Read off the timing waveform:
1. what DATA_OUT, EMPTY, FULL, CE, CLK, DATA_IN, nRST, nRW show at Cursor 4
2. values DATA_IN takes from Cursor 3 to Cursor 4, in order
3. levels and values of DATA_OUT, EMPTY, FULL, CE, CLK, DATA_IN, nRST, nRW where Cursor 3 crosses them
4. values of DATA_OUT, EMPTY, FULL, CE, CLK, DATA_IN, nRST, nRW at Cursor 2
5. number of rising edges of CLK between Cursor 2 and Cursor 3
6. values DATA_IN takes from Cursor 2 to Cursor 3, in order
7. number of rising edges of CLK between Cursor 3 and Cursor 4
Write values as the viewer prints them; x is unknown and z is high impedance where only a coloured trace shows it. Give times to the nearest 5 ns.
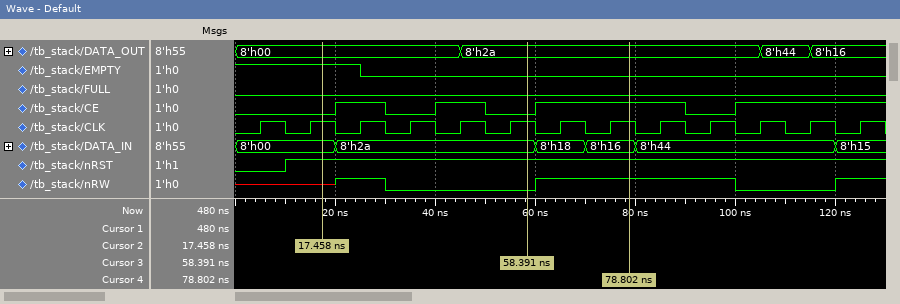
DATA_OUT=8'h2a, EMPTY=0, FULL=0, CE=1, CLK=1, DATA_IN=8'h16, nRST=1, nRW=1
8'h2a, 8'h18, 8'h16
DATA_OUT=8'h2a, EMPTY=0, FULL=0, CE=0, CLK=1, DATA_IN=8'h2a, nRST=1, nRW=0
DATA_OUT=8'h00, EMPTY=1, FULL=0, CE=0, CLK=1, DATA_IN=8'h00, nRST=1, nRW=x
4
8'h00, 8'h2a
2
